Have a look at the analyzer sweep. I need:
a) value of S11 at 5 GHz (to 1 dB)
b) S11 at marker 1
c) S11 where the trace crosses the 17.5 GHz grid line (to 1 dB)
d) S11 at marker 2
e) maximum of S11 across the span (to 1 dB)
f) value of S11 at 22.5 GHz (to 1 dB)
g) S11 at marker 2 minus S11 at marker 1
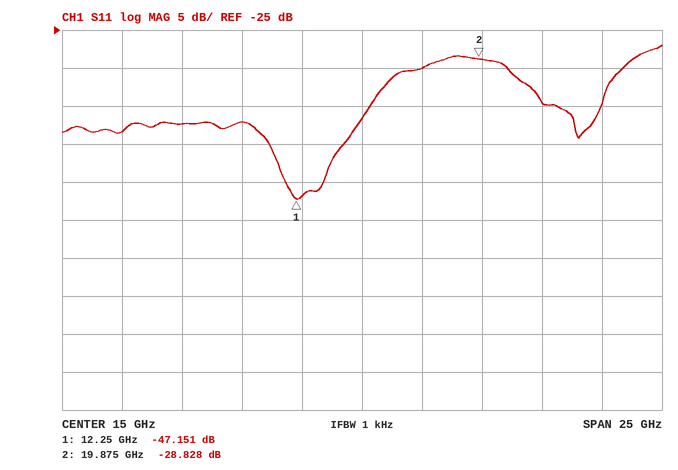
-38 dB
-47.151 dB
-30 dB
-28.828 dB
-27 dB
-35 dB
18.323 dB
